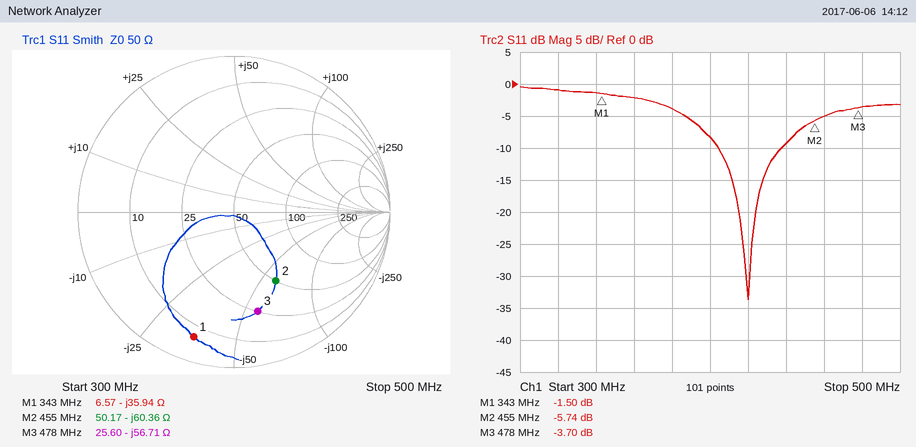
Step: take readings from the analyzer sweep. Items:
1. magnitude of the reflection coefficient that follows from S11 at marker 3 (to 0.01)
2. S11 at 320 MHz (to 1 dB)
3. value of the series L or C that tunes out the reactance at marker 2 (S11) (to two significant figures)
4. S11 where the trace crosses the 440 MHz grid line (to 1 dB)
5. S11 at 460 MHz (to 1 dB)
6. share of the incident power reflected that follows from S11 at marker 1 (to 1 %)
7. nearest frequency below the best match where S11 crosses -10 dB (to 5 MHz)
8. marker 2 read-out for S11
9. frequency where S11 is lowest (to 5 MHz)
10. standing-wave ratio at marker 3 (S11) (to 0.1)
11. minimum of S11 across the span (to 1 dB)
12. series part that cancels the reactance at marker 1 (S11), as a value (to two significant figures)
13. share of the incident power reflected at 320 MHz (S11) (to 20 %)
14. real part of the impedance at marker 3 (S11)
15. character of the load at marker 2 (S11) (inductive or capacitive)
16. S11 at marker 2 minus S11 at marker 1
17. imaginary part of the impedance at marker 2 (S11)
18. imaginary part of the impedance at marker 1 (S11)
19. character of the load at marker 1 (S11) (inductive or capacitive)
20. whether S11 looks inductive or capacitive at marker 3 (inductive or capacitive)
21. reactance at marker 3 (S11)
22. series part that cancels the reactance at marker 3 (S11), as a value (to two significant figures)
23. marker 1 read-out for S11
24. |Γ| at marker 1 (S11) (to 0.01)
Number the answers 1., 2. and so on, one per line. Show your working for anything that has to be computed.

1. 10^(-3.7/20) ≈ 0.65
2. -1 dB
3. L = 60.36 Ω/(2π × 455 MHz) ≈ 21 nH
4. -9 dB
5. -5 dB
6. 10^(-1.5/10) ≈ 71 %
7. 405 MHz
8. -5.74 dB
9. 420 MHz
10. 4.8
11. -34 dB
12. L = 35.94 Ω/(2π × 343 MHz) ≈ 17 nH
13. 10^(-1/10) ≈ 79.4 %, so 80 % to the nearest 20 %
14. 25.60 Ω
15. capacitive
16. -5.74 − (-1.5) = -4.24 dB
17. -60.36 Ω
18. -35.94 Ω
19. capacitive
20. capacitive
21. -56.71 Ω
22. L = 56.71 Ω/(2π × 478 MHz) ≈ 19 nH
23. -1.50 dB
24. 0.84
